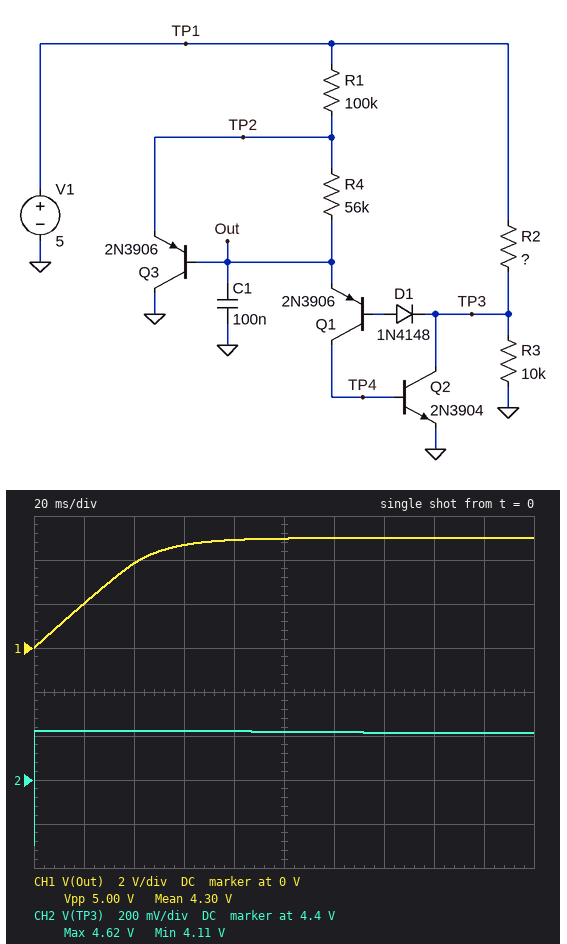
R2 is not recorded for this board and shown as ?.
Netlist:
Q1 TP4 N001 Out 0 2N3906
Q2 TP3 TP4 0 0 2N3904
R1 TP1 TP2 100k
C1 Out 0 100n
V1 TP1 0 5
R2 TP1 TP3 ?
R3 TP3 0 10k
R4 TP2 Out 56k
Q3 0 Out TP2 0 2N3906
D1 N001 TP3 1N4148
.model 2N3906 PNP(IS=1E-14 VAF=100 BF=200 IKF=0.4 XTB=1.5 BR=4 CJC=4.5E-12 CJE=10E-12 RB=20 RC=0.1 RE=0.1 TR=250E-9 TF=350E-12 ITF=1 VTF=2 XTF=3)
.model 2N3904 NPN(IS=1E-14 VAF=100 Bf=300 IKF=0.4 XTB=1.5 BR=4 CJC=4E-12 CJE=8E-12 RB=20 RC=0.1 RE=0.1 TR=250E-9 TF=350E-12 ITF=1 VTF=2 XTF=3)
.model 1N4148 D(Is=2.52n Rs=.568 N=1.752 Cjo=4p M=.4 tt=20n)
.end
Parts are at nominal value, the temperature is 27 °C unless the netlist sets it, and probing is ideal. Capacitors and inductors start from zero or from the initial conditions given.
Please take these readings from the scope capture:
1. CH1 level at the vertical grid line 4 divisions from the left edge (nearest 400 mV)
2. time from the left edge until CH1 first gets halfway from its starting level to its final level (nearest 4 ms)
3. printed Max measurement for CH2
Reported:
4.8 V
24 ms
4.62 V
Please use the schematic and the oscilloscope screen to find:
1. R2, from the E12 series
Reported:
820 Ω
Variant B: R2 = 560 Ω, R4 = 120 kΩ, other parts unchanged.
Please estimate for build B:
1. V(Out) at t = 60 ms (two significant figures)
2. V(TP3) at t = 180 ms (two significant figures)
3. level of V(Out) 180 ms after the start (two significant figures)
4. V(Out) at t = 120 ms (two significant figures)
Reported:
2.9 V
4.7 V
5.0 V
4.8 V
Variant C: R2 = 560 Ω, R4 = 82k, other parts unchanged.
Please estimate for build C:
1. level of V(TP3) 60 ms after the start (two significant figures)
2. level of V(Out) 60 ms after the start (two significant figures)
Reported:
4.7 V
4.0 V
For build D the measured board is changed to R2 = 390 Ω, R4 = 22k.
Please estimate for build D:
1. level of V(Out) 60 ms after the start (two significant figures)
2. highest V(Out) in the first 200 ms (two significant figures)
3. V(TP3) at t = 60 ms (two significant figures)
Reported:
5.0 V
5.0 V
4.8 V
